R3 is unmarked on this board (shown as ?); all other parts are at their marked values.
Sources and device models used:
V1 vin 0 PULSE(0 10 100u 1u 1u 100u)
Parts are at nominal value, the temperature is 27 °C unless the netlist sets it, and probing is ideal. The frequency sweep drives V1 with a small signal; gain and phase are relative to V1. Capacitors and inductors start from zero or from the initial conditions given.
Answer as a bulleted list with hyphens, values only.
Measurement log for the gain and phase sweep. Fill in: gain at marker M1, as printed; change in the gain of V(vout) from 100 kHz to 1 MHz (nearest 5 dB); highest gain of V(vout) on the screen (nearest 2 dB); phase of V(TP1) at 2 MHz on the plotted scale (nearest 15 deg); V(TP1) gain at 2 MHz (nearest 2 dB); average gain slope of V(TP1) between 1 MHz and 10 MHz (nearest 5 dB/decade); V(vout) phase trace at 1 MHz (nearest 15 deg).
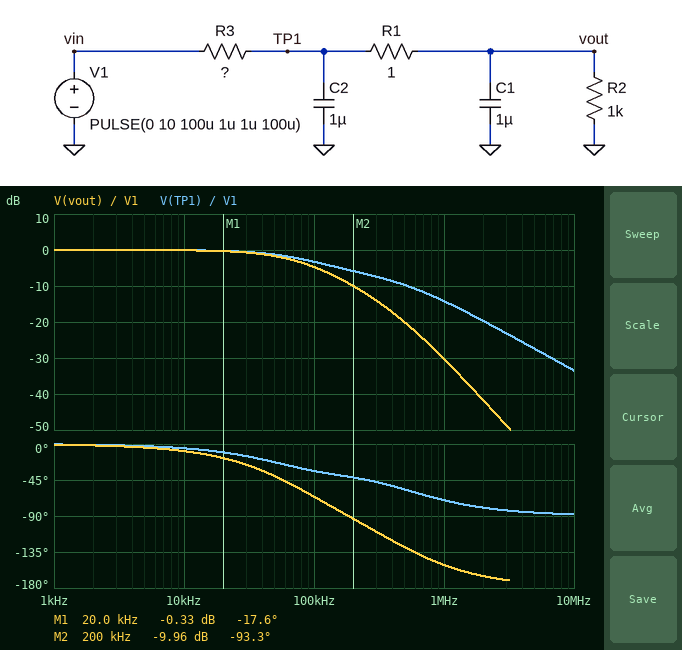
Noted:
- -0.33 dB
- -25 dB
- 0 dB
- -75 deg
- -20 dB
- -20 dB/decade
- -150 deg
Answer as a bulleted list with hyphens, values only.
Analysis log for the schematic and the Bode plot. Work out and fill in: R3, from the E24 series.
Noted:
- 0.75 Ω
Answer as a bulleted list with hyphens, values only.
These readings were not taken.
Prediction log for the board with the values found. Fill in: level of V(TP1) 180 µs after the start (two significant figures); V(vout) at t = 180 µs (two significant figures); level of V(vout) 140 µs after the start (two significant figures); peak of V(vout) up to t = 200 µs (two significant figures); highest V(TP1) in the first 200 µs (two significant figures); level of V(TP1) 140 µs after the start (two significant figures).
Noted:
- 10 V
- 10 V
- 10 V
- 10 V
- 10 V
- 10 V
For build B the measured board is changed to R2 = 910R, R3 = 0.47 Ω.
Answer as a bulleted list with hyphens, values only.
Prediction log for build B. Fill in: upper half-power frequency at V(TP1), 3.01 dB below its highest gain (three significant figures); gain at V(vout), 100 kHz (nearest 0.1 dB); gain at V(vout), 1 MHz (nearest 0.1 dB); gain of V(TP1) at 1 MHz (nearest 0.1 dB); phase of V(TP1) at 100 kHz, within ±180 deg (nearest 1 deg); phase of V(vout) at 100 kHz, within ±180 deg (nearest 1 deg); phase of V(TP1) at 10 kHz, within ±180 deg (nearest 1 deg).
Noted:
- 157 kHz
- -3.3 dB
- -26.6 dB
- -10.5 dB
- -24 deg
- -56 deg
- -3 deg
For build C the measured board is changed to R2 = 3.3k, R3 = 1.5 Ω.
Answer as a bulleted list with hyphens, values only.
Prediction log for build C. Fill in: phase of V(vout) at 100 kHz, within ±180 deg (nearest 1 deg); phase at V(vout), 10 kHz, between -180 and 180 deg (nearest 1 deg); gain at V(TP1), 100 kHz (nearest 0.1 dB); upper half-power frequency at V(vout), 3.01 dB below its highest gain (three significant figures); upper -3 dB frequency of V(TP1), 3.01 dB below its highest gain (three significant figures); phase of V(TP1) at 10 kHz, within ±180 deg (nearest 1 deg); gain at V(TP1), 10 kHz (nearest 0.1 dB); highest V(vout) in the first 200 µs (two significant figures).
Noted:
- -81 deg
- -14 deg
- -6.7 dB
- 43.9 kHz
- 47.6 kHz
- -11 deg
- -0.2 dB
- 10 V
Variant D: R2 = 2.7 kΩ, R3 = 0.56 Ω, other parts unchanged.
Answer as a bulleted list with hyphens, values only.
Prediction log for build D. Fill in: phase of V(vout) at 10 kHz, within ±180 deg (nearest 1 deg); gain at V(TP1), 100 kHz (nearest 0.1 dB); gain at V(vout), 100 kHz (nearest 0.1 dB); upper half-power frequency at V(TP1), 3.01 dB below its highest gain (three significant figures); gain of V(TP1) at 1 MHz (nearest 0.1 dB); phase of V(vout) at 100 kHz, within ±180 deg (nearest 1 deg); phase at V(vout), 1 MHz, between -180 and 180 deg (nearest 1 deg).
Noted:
- -8 deg
- -2.3 dB
- -3.8 dB
- 127 kHz
- -11.9 dB
- -60 deg
- -148 deg
